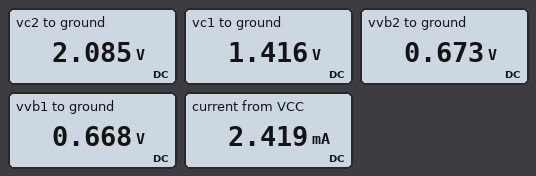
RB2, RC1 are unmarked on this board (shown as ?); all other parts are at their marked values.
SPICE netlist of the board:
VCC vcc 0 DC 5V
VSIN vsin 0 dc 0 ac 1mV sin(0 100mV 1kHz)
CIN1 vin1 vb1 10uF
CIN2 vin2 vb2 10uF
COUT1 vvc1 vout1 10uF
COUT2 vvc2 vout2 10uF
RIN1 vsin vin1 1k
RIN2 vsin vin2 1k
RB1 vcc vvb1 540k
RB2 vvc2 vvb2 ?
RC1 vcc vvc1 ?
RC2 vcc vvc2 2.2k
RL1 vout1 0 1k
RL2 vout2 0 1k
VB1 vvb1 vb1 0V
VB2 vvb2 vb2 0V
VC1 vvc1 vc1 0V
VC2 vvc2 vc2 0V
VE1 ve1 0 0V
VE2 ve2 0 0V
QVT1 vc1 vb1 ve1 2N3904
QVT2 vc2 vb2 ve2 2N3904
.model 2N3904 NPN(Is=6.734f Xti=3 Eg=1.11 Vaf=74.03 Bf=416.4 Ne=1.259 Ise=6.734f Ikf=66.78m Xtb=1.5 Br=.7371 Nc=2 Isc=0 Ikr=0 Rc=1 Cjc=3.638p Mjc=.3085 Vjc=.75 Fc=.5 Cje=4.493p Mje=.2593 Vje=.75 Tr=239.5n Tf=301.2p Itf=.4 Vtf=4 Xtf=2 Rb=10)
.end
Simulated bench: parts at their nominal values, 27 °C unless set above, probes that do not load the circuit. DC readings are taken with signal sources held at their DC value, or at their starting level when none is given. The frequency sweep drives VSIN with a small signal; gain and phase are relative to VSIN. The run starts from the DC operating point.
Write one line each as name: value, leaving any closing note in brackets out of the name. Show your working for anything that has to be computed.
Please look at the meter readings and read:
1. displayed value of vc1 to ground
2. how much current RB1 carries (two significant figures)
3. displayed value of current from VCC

displayed value of vc1 to ground: 1.416 V
how much current RB1 carries: (5 V - 668 mV) / 540 kΩ = 8.0 µA
displayed value of current from VCC: 2.419 mA
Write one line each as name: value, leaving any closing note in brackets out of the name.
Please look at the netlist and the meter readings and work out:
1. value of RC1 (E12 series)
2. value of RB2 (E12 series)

value of RC1: 3.3 kΩ
value of RB2: 150 kΩ
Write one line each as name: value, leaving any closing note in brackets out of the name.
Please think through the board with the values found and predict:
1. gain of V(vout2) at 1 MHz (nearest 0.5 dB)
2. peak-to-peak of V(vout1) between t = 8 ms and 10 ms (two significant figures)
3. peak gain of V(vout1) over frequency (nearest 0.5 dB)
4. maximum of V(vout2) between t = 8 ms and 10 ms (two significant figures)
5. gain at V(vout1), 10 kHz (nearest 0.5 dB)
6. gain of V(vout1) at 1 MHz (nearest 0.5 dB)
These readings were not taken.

gain of V(vout2) at 1 MHz: 26.0 dB
peak-to-peak of V(vout1) between t = 8 ms and 10 ms: 2.0 V
peak gain of V(vout1) over frequency: 28.0 dB
maximum of V(vout2) between t = 8 ms and 10 ms: 960 mV
gain at V(vout1), 10 kHz: 28.0 dB
gain of V(vout1) at 1 MHz: 26.5 dB
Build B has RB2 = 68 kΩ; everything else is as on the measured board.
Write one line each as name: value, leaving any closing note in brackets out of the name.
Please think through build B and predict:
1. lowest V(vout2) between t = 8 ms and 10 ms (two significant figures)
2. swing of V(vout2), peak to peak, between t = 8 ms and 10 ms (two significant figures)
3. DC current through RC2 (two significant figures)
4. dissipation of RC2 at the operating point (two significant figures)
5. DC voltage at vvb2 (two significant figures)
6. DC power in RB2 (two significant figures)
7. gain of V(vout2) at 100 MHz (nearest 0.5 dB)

lowest V(vout2) between t = 8 ms and 10 ms: -1.2 V
swing of V(vout2), peak to peak, between t = 8 ms and 10 ms: 2.3 V
DC current through RC2: 1.6 mA
dissipation of RC2 at the operating point: 5.7 mW
DC voltage at vvb2: 680 mV
DC power in RB2: 8.7 µW
gain of V(vout2) at 100 MHz: -7.5 dB
